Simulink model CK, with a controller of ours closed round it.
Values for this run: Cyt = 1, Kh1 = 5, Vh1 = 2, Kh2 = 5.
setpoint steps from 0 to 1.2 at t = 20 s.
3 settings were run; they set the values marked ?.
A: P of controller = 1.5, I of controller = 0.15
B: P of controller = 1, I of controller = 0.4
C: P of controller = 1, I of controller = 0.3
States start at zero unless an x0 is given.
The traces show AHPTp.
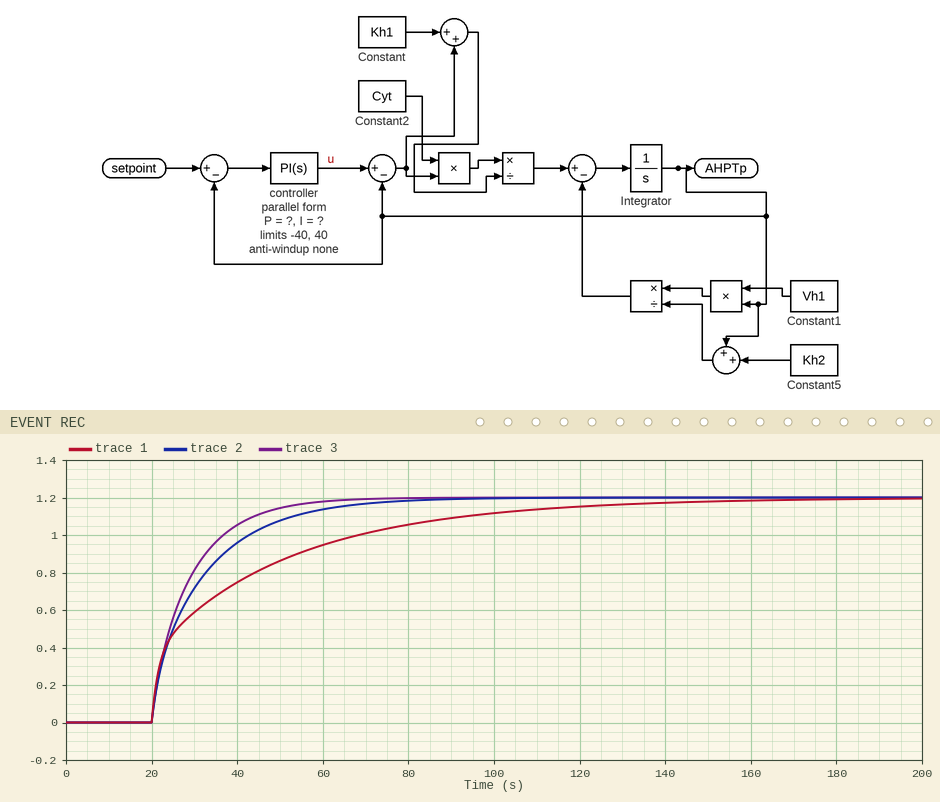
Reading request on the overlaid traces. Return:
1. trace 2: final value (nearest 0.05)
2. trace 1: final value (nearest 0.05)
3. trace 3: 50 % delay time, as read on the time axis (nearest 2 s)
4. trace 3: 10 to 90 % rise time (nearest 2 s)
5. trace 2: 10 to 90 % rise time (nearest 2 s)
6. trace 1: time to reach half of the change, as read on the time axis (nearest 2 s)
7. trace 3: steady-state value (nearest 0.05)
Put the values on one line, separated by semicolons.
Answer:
1.20; 1.20; 26 s; 22 s; 30 s; 30 s; 1.20
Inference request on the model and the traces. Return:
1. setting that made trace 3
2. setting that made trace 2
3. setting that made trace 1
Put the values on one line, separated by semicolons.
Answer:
B; C; A
